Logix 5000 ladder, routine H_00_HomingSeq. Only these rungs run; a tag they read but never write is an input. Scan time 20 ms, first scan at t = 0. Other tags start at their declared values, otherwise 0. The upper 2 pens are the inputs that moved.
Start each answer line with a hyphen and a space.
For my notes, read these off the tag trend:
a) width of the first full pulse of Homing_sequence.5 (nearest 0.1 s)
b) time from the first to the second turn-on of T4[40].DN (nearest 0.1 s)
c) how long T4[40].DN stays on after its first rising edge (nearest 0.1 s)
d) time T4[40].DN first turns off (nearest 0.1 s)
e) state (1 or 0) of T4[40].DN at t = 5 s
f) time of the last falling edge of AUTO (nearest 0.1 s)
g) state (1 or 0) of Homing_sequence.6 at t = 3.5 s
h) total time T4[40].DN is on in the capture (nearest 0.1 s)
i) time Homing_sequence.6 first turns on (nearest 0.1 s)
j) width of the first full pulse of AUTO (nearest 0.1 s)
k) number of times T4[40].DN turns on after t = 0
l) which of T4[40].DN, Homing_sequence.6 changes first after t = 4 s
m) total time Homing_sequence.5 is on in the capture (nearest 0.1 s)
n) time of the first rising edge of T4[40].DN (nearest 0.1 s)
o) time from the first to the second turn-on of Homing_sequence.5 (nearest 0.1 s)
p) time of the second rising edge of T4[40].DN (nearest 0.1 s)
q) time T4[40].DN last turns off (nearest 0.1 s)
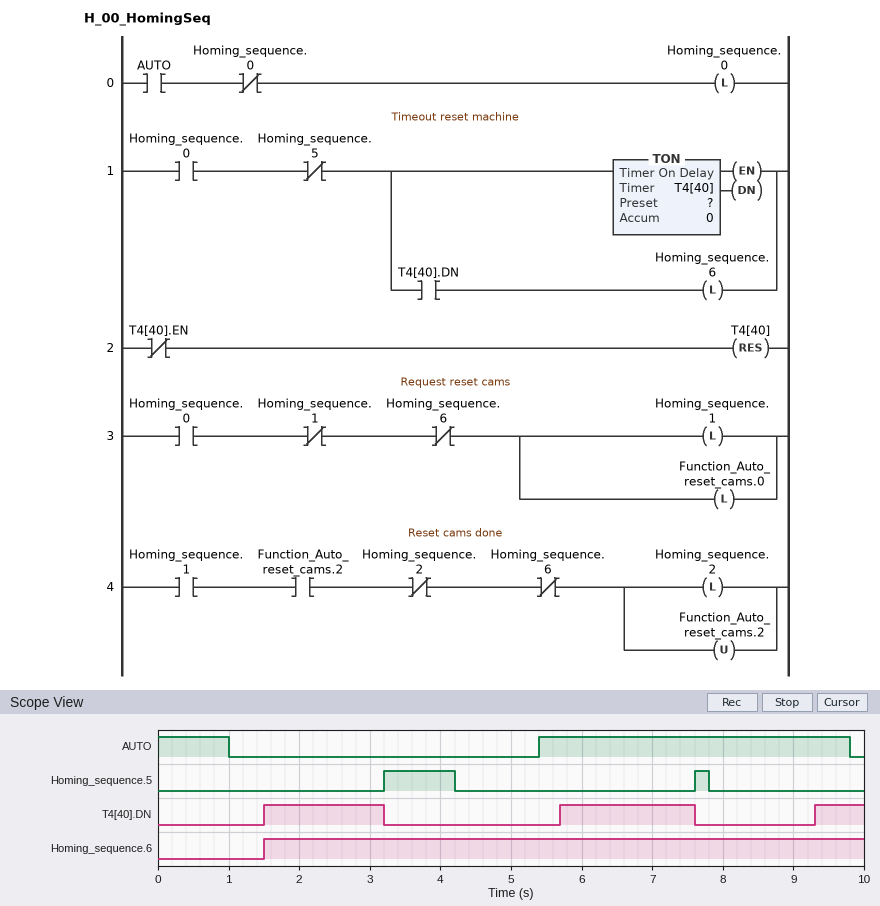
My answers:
- 1.0 s
- 4.2 s
- 1.7 s
- 3.2 s
- 0
- 9.8 s
- 1
- 4.3 s
- 1.5 s
- 4.4 s
- 3
- T4[40].DN
- 1.2 s
- 1.5 s
- 4.4 s
- 5.7 s
- 7.6 s
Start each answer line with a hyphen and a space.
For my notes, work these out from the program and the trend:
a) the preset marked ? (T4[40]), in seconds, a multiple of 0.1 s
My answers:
- 1.5 s
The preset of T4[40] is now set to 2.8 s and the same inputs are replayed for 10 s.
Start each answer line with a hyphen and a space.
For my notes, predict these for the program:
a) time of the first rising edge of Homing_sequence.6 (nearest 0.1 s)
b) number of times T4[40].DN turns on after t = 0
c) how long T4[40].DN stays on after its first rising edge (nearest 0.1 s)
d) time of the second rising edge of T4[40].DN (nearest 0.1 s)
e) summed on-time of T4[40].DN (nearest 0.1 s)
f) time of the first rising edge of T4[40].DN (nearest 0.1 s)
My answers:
- 2.8 s
- 2
- 0.4 s
- 7.0 s
- 1.0 s
- 2.8 s
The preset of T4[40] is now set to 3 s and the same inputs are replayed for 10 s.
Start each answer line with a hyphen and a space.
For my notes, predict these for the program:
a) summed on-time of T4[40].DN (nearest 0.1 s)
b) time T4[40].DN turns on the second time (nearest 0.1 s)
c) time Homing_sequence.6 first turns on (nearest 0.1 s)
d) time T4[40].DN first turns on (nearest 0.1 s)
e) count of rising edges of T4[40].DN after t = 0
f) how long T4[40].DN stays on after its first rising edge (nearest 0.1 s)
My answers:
- 0.6 s
- 7.2 s
- 3.0 s
- 3.0 s
- 2
- 0.2 s
